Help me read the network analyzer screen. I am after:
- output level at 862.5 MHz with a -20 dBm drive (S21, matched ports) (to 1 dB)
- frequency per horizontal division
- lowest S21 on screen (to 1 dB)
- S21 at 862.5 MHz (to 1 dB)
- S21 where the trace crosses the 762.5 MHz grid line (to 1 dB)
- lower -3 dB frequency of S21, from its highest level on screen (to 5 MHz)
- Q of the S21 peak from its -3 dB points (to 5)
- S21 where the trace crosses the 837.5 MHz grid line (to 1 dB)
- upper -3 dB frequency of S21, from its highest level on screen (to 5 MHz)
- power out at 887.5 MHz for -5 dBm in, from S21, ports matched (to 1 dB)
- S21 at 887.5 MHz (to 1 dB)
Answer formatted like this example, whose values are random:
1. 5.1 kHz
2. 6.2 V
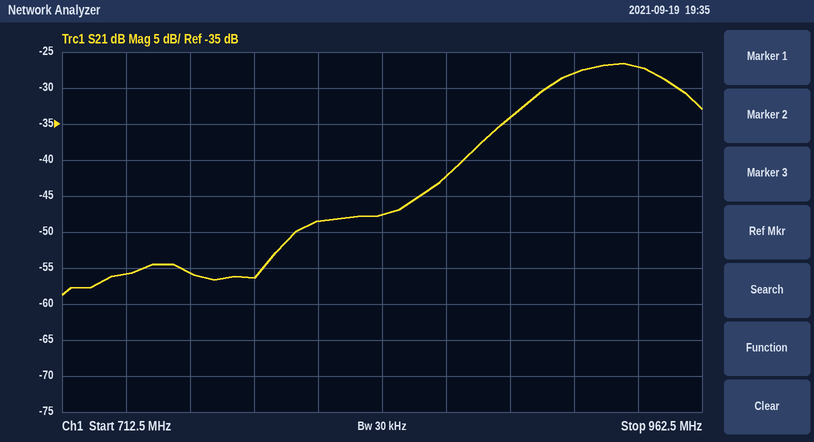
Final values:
1. -62 dBm
2. 25 MHz
3. -59 dB
4. -42 dB
5. -56 dB
6. 905 MHz
7. 20
8. -48 dB
9. 950 MHz
10. -39 dBm
11. -34 dB
